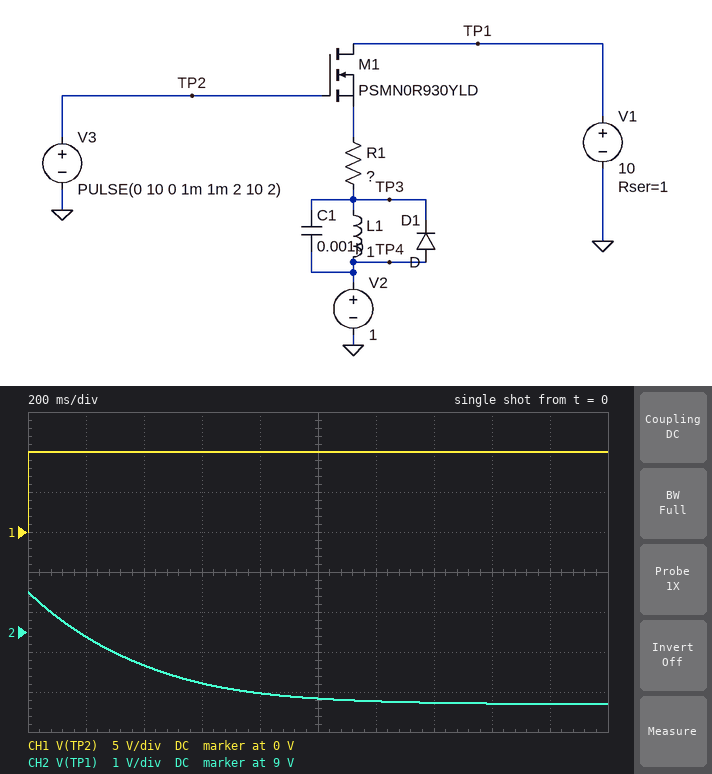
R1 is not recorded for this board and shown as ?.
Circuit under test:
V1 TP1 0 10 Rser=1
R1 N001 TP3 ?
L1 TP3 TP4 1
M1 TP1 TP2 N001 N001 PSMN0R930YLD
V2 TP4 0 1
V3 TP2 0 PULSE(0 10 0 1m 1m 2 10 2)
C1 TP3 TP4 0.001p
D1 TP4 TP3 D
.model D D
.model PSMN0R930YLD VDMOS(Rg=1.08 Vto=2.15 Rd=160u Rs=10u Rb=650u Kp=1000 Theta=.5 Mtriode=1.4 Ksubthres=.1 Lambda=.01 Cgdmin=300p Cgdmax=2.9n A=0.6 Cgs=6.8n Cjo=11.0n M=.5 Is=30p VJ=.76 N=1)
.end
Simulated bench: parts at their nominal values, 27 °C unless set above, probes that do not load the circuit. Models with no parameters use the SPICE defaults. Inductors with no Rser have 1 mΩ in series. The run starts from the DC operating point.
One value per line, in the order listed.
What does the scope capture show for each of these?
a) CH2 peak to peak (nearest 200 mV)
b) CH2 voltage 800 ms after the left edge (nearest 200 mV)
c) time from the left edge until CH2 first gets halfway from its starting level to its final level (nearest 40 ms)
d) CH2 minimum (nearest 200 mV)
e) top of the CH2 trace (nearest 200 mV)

2.8 V
7.4 V
280 ms
7.2 V
10.0 V
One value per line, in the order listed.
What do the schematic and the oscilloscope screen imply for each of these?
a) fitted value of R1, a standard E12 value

2.2 Ω
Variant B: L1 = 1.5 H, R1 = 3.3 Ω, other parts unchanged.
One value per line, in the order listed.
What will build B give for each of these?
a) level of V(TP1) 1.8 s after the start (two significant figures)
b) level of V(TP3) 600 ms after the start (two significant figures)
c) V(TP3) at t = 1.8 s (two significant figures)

8.0 V
2.8 V
1.1 V
